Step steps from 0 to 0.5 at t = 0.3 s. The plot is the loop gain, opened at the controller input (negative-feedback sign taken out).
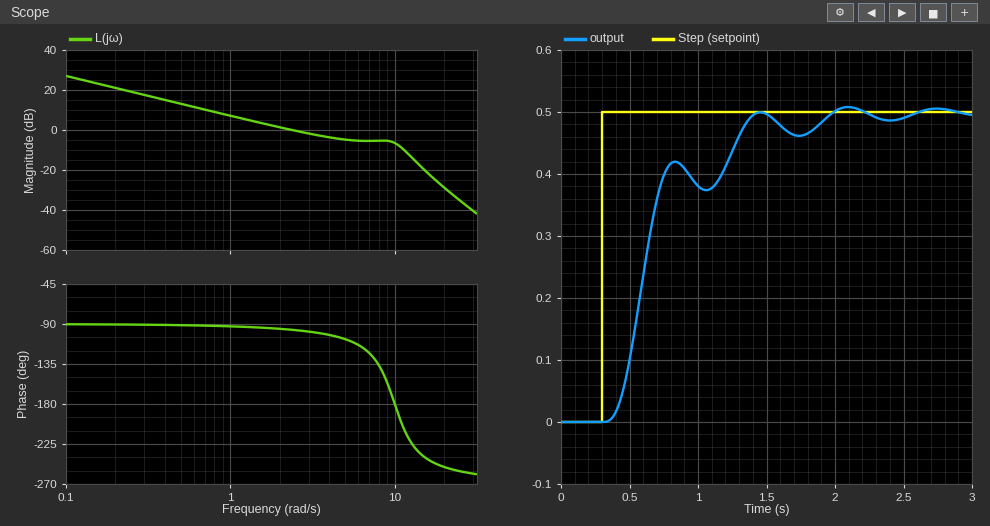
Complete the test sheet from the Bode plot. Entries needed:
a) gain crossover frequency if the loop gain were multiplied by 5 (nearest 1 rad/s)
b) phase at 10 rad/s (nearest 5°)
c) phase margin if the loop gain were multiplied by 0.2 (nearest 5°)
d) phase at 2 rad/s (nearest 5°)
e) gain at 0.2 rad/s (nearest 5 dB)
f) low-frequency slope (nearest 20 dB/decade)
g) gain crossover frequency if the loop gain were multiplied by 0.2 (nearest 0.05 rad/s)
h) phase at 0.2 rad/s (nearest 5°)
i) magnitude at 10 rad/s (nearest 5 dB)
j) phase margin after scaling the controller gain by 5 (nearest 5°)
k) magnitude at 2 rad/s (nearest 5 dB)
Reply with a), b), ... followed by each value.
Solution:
a) 13 rad/s
b) -180°
c) 90°
d) -95°
e) 20 dB
f) -20 dB/decade
g) 0.45 rad/s
h) -90°
i) -5 dB
j) -45°
k) 0 dB
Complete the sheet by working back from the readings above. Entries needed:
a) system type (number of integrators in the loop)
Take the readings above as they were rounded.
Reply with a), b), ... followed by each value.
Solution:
a) 1
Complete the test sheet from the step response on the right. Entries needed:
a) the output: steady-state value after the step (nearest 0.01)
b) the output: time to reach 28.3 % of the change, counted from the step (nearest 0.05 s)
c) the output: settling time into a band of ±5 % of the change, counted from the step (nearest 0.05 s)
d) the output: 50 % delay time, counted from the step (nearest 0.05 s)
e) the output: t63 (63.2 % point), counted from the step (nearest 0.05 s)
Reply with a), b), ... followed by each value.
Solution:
a) 0.50
b) 0.25 s
c) 1.55 s
d) 0.30 s
e) 0.35 s
